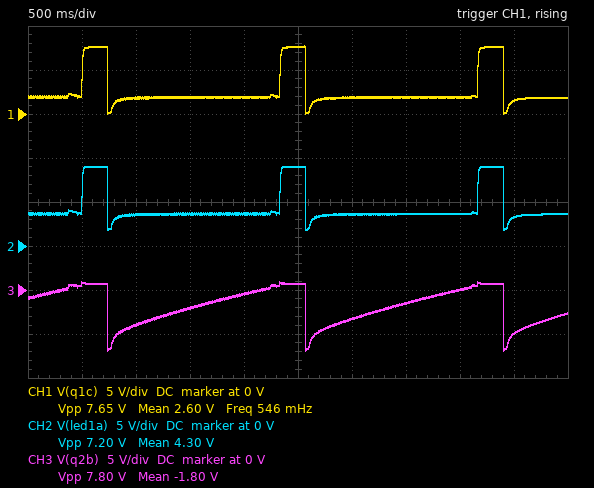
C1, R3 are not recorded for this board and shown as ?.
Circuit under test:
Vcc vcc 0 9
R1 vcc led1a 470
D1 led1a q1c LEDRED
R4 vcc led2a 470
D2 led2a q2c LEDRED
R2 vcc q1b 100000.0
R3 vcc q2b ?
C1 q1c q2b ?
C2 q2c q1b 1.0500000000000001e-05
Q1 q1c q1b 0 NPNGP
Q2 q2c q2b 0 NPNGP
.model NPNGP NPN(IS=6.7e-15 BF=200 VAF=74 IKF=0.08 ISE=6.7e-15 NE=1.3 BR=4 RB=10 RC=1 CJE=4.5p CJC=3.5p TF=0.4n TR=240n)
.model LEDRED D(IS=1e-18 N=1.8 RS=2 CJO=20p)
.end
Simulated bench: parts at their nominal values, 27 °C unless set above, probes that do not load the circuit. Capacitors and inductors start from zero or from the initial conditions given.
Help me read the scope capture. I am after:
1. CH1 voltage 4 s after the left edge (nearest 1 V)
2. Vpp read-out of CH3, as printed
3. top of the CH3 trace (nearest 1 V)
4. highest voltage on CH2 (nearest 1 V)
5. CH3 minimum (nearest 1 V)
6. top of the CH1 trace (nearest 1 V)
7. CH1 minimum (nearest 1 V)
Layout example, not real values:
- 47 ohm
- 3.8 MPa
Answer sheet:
- 2 V
- 7.80 V
- 1 V
- 9 V
- -7 V
- 8 V
- 0 V
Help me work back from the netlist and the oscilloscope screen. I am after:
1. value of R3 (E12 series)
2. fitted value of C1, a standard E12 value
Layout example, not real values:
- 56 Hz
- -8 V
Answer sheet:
- 270 kΩ
- 12 µF
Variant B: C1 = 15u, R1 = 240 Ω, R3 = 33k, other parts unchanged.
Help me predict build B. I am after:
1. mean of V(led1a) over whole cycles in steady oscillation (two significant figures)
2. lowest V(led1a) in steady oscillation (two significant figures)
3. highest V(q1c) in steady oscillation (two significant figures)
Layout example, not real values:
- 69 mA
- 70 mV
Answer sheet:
- 8.3 V
- 1.9 V
- 7.7 V
